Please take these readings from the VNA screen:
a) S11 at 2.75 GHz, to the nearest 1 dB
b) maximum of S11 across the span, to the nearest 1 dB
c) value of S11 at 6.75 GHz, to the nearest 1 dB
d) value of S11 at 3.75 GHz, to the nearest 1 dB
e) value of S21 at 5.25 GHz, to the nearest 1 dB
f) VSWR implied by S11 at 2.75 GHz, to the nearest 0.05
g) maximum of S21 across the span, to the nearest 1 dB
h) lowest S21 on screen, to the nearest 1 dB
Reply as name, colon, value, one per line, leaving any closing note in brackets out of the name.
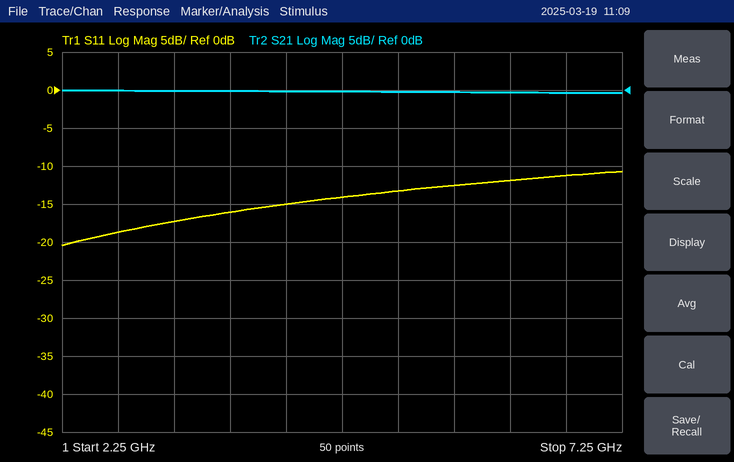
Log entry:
S11 at 2.75 GHz, to the nearest 1 dB: -19 dB
maximum of S11 across the span, to the nearest 1 dB: -11 dB
value of S11 at 6.75 GHz, to the nearest 1 dB: -11 dB
value of S11 at 3.75 GHz, to the nearest 1 dB: -16 dB
value of S21 at 5.25 GHz, to the nearest 1 dB: 0 dB
VSWR implied by S11 at 2.75 GHz, to the nearest 0.05: 1.25
maximum of S21 across the span, to the nearest 1 dB: 0 dB
lowest S21 on screen, to the nearest 1 dB: 0 dB
